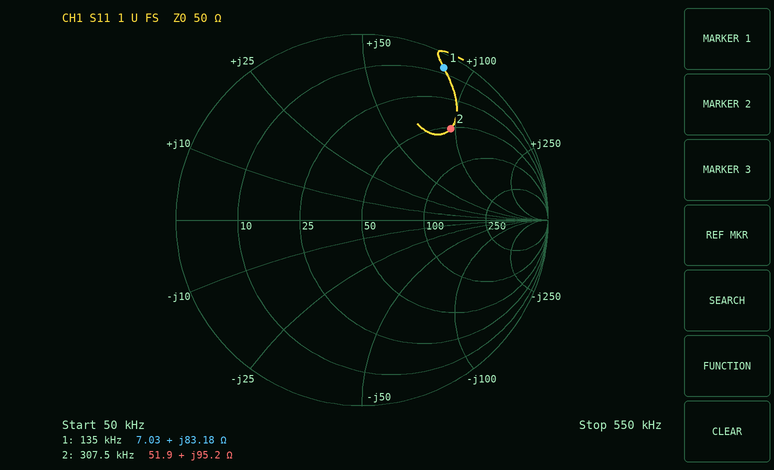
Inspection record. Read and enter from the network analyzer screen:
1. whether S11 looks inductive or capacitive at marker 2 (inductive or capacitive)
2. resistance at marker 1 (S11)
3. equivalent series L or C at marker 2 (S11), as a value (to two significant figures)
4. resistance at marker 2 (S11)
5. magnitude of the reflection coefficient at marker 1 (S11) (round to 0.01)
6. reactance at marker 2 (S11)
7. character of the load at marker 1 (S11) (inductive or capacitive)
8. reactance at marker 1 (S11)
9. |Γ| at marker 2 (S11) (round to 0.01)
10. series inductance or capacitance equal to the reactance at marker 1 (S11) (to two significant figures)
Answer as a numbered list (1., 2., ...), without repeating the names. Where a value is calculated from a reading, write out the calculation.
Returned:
1. inductive
2. 7.03 Ω
3. L = 95.2 Ω/(2π × 307.5 kHz) ≈ 49 µH
4. 51.9 Ω
5. 0.93
6. +95.2 Ω
7. inductive
8. +83.18 Ω
9. 0.68
10. L = 83.18 Ω/(2π × 135 kHz) ≈ 98 µH
